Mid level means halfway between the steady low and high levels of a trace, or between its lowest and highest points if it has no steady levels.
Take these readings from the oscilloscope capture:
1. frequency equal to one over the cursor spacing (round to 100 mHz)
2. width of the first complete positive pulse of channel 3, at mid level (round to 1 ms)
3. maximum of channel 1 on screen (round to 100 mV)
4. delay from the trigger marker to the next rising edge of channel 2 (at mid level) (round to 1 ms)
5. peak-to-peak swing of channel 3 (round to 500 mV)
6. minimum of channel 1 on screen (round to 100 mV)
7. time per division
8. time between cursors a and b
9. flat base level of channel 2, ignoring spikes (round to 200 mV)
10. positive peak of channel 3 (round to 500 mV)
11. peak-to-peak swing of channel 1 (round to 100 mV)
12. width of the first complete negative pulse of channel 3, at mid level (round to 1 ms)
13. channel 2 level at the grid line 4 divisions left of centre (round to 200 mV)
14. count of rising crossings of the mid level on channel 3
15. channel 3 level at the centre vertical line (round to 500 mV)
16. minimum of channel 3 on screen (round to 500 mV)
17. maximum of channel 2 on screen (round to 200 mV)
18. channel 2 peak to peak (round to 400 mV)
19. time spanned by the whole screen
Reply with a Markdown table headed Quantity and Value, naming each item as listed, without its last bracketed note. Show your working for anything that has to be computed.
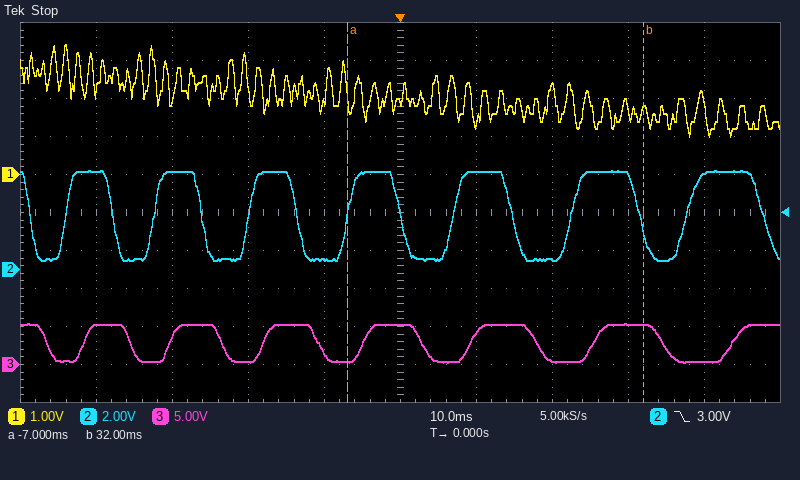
| Quantity | Value |
|---|---|
| frequency equal to one over the cursor spacing | 1 / 39 ms ≈ 25.6 Hz |
| width of the first complete positive pulse of channel 3, at mid level | 6 ms |
| maximum of channel 1 on screen | 3.4 V |
| delay from the trigger marker to the next rising edge of channel 2 (at mid level) | 7 ms |
| peak-to-peak swing of channel 3 | 5.5 V − (500 mV) = 5.0 V |
| minimum of channel 1 on screen | 1.0 V |
| time per division | 10 ms |
| time between cursors a and b | 32 ms − (-7 ms) = 39 ms |
| flat base level of channel 2, ignoring spikes | 600 mV |
| positive peak of channel 3 | 5.5 V |
| peak-to-peak swing of channel 1 | 3.4 V − (1.0 V) = 2.4 V |
| width of the first complete negative pulse of channel 3, at mid level | 5 ms |
| channel 2 level at the grid line 4 divisions left of centre | 5.2 V |
| count of rising crossings of the mid level on channel 3 | 7 |
| channel 3 level at the centre vertical line | 5.5 V |
| minimum of channel 3 on screen | 500 mV |
| maximum of channel 2 on screen | 5.2 V |
| channel 2 peak to peak | 4.8 V |
| time spanned by the whole screen | 100 ms |
